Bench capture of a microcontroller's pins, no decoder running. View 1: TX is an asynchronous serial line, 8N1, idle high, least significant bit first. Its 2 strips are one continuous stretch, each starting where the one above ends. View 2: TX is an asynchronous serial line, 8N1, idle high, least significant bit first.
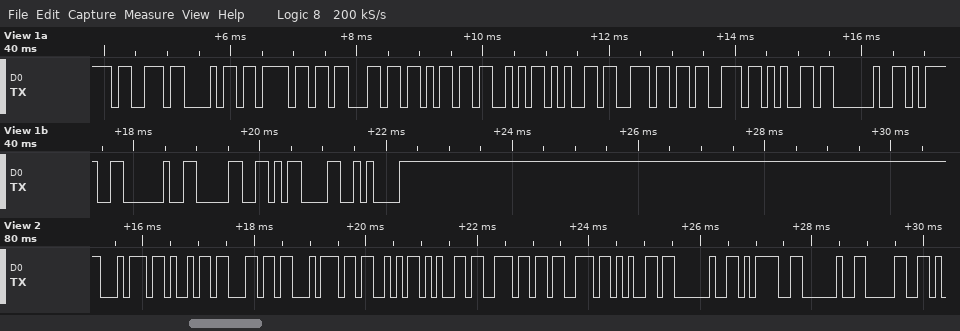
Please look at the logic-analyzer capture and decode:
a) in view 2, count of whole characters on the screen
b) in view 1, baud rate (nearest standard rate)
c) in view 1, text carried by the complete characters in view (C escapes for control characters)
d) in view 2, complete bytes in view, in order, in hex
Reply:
13
9600 baud
"shockSense = 0\r\n"
0x74 0x69 0x6C 0x74 0x53 0x65 0x6E 0x73 0x65 0x20 0x3D 0x20 0x30
